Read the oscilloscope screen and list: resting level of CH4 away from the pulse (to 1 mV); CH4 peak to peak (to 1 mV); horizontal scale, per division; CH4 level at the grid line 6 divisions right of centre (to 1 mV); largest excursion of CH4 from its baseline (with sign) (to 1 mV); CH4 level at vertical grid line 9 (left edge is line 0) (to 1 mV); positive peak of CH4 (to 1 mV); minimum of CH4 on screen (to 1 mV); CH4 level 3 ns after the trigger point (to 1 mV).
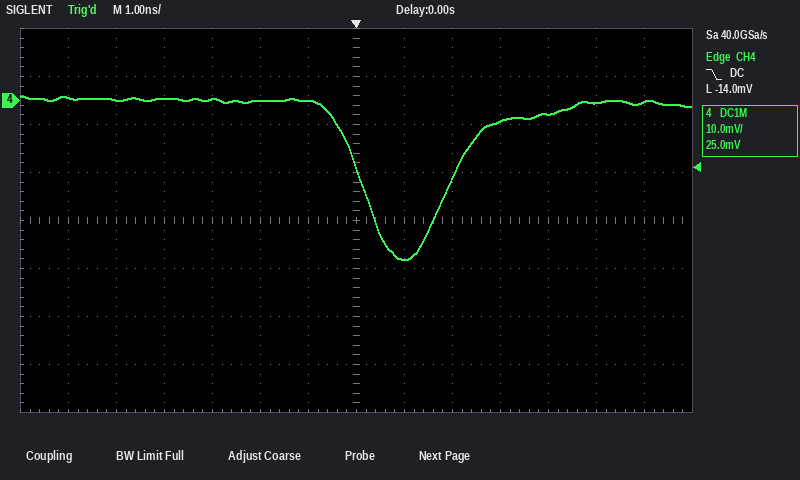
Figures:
0 mV
34 mV
1 ns
0 mV
-33 mV
-16 mV
1 mV
-33 mV
-4 mV
